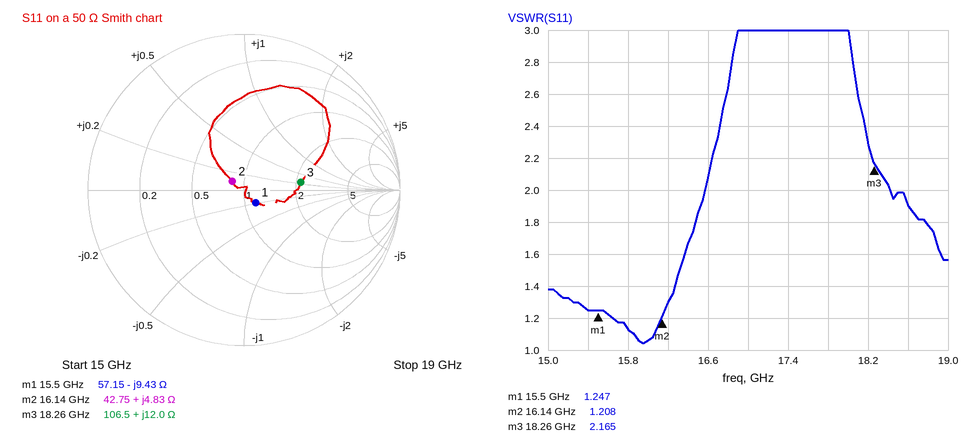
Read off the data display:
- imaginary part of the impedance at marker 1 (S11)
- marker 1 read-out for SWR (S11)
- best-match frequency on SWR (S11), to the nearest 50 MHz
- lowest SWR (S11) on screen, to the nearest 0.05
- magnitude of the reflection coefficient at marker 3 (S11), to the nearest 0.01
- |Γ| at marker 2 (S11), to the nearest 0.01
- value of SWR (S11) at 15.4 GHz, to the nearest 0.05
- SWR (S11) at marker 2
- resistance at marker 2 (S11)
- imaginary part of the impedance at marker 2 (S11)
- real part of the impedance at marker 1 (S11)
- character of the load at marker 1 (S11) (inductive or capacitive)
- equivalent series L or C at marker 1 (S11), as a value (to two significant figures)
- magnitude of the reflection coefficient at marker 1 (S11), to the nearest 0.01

-9.43 Ω
1.247
15.95 GHz
1.05
0.37
0.09
1.25
1.208
42.75 Ω
+4.83 Ω
57.15 Ω
capacitive
1.1 pF
0.11
